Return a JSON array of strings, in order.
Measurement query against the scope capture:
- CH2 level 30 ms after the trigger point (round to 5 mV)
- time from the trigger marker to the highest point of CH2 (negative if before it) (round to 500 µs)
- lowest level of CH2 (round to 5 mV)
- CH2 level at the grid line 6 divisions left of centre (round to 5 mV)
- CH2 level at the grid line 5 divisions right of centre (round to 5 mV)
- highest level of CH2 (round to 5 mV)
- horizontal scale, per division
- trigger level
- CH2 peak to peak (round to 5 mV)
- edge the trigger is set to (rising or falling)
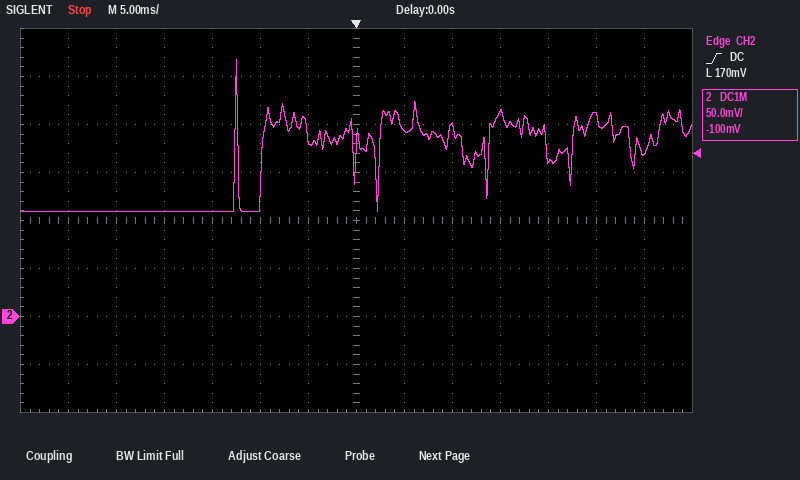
["170 mV", "-12.5 ms", "110 mV", "110 mV", "210 mV", "270 mV", "5 ms", "170 mV", "160 mV", "rising"]
